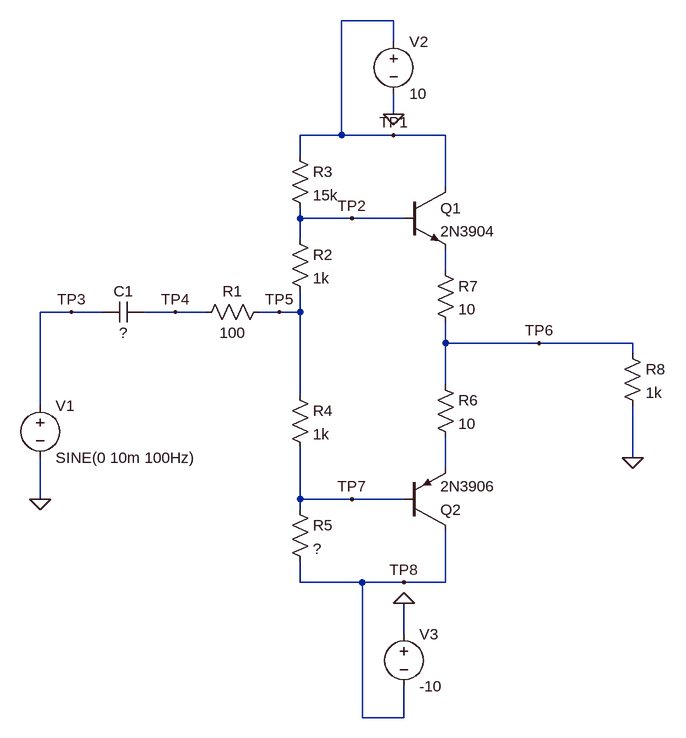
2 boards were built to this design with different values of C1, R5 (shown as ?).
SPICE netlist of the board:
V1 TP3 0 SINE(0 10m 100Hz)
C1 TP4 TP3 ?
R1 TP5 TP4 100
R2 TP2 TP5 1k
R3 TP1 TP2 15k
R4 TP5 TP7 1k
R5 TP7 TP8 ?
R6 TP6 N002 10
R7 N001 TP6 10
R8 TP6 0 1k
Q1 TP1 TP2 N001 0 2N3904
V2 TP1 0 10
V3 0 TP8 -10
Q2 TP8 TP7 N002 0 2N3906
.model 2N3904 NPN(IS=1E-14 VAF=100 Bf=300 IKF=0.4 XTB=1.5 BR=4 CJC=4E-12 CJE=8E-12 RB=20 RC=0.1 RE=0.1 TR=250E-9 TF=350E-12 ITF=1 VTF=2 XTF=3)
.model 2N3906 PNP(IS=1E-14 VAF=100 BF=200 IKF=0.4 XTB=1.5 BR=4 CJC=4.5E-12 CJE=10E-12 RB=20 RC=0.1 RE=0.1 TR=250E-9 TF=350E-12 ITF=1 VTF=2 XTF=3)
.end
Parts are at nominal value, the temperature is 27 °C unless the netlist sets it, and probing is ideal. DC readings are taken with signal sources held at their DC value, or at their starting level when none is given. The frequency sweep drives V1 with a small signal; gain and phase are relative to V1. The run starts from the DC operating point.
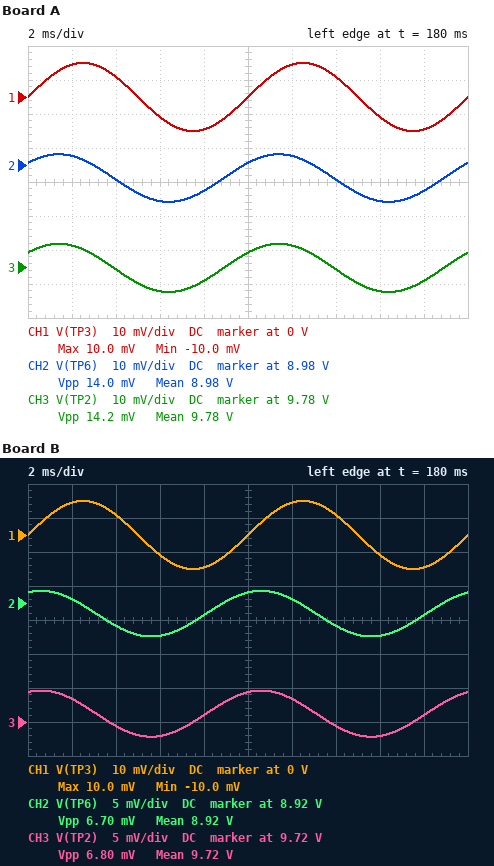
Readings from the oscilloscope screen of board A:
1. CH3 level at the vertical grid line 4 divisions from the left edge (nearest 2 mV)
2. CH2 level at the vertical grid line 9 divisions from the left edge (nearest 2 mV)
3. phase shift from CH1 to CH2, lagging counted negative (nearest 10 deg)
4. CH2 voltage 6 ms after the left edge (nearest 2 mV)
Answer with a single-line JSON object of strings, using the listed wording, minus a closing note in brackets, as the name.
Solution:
{"CH3 level at the vertical grid line 4 divisions from the left edge": "9.776 V", "CH2 level at the vertical grid line 9 divisions from the left edge": "8.972 V", "phase shift from CH1 to CH2, lagging counted negative": "40 deg", "CH2 voltage 6 ms after the left edge": "8.970 V"}
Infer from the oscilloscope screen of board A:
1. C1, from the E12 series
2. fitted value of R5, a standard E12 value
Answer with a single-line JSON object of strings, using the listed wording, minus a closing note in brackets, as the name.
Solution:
{"C1, from the E12 series": "270 nF", "fitted value of R5, a standard E12 value": "12 kΩ"}
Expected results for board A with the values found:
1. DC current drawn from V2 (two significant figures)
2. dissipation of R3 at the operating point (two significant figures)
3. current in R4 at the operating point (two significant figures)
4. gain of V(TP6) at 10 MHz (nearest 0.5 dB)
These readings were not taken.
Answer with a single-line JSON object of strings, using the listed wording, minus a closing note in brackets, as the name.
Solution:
{"DC current drawn from V2": "9.0 mA", "dissipation of R3 at the operating point": "3.2 µW", "current in R4 at the operating point": "16 µA", "gain of V(TP6) at 10 MHz": "-1.0 dB"}
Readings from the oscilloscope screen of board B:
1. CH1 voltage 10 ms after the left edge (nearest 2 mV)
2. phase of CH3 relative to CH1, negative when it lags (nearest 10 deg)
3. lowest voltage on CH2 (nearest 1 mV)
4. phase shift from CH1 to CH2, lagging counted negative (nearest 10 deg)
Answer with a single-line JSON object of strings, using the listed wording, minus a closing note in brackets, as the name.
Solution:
{"CH1 voltage 10 ms after the left edge": "0 V", "phase of CH3 relative to CH1, negative when it lags": "70 deg", "lowest voltage on CH2": "8.915 V", "phase shift from CH1 to CH2, lagging counted negative": "70 deg"}
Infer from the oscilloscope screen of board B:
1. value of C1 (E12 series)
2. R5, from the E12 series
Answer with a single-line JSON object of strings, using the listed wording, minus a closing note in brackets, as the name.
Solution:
{"value of C1": "68 nF", "R5, from the E12 series": "22 kΩ"}
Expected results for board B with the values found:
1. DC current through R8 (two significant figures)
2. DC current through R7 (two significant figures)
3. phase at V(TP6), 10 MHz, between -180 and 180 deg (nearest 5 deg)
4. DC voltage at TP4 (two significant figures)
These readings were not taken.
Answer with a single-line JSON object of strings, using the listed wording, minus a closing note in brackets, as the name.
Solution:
{"DC current through R8": "8.9 mA", "DC current through R7": "8.9 mA", "phase at V(TP6), 10 MHz, between -180 and 180 deg": "-15 deg", "DC voltage at TP4": "9.7 V"}
